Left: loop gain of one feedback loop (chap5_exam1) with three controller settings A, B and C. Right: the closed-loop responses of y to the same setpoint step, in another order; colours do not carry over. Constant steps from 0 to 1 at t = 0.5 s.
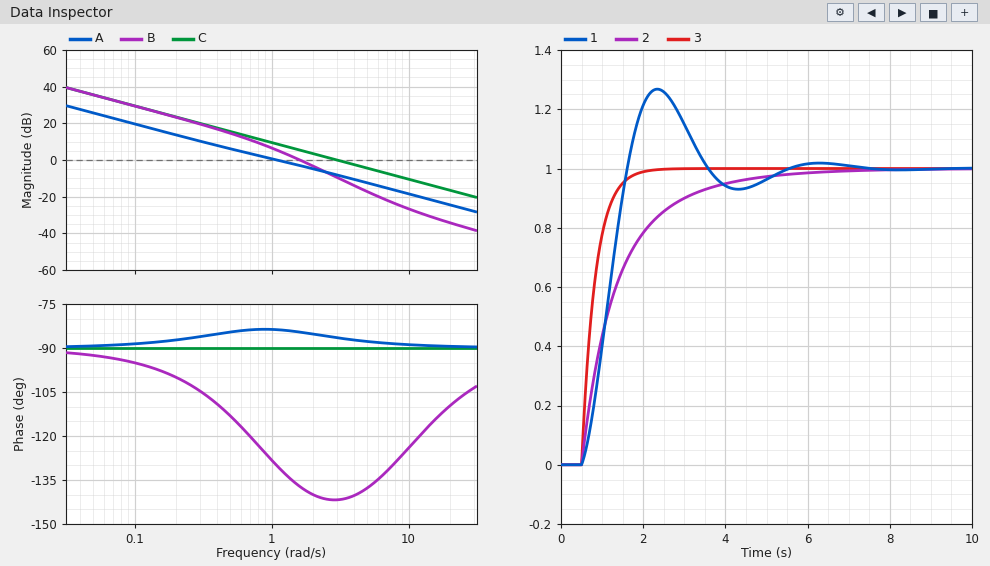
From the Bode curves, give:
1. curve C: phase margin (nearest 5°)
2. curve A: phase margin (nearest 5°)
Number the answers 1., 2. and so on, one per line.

1. 90°
2. 95°
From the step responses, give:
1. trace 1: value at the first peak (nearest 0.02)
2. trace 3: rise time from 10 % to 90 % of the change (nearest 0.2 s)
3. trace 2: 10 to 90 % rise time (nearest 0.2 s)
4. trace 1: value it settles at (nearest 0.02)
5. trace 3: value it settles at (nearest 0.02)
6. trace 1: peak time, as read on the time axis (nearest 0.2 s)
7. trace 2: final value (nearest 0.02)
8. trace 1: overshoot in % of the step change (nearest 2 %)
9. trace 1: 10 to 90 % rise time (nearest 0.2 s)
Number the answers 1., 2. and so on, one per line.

1. 1.26
2. 0.8 s
3. 2.4 s
4. 1.00
5. 1.00
6. 2.4 s
7. 1.00
8. 26 %
9. 0.8 s
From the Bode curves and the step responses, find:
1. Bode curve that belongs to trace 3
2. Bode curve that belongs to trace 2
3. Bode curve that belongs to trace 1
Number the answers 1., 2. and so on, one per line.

1. C
2. A
3. B
